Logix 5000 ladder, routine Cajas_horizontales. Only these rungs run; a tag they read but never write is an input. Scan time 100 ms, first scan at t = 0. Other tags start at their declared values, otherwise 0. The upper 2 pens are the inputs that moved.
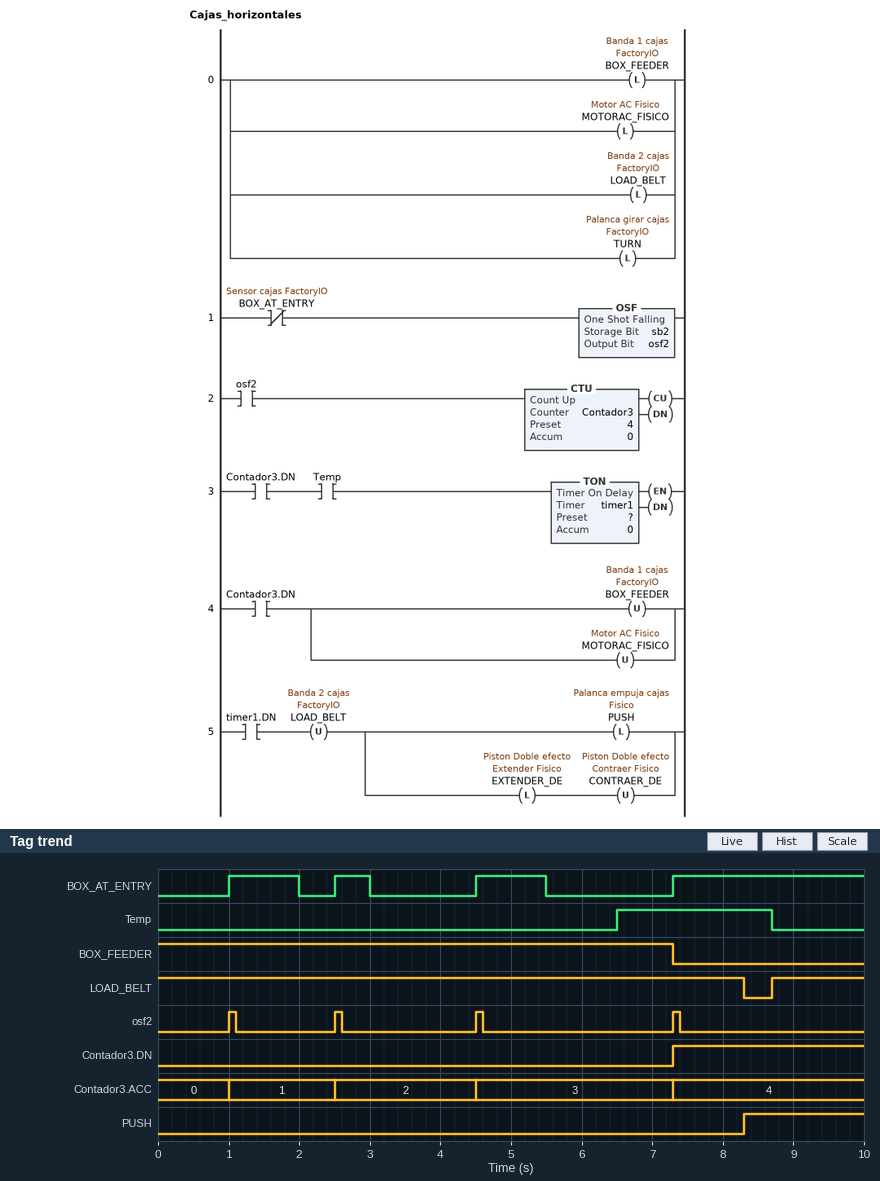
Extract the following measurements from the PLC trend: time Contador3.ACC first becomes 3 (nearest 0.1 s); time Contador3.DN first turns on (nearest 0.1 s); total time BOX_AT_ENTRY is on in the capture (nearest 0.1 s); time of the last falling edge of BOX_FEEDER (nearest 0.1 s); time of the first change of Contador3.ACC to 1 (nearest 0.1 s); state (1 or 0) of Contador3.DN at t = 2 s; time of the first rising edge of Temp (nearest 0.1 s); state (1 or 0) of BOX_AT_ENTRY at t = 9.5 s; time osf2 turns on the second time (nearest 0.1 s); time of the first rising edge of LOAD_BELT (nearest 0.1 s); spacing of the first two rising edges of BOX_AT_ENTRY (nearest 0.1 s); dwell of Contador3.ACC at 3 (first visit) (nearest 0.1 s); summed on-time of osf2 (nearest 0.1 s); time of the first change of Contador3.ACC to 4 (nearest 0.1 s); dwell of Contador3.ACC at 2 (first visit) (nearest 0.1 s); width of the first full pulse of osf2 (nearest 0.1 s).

4.5 s
7.3 s
5.2 s
7.3 s
1.0 s
0
6.5 s
1
2.5 s
8.7 s
1.5 s
2.8 s
0.4 s
7.3 s
2.0 s
0.1 s
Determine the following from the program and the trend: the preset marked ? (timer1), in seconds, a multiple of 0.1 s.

1.0 s
